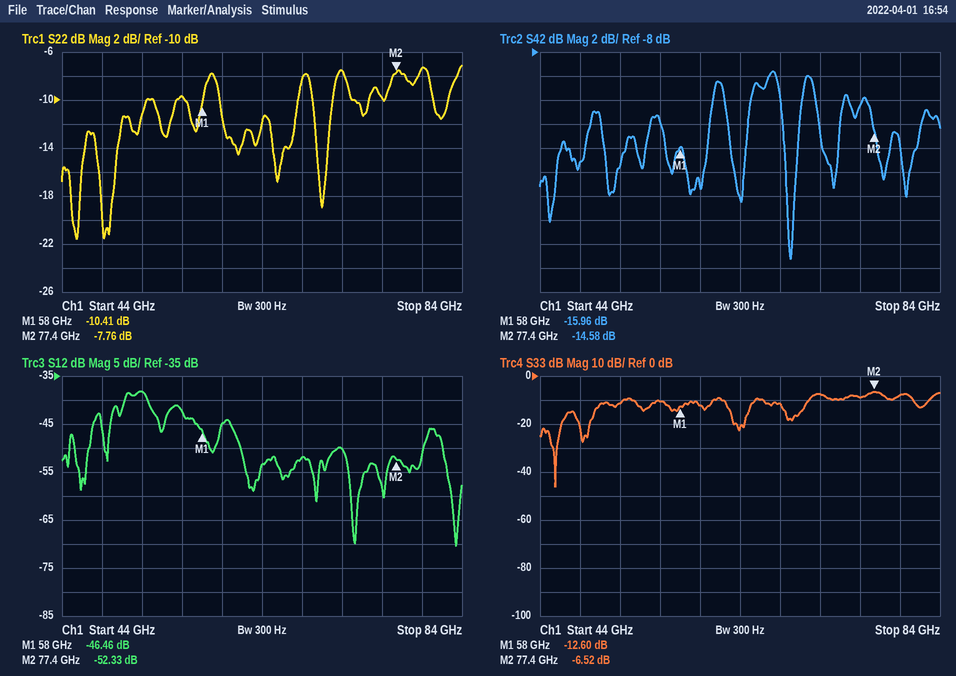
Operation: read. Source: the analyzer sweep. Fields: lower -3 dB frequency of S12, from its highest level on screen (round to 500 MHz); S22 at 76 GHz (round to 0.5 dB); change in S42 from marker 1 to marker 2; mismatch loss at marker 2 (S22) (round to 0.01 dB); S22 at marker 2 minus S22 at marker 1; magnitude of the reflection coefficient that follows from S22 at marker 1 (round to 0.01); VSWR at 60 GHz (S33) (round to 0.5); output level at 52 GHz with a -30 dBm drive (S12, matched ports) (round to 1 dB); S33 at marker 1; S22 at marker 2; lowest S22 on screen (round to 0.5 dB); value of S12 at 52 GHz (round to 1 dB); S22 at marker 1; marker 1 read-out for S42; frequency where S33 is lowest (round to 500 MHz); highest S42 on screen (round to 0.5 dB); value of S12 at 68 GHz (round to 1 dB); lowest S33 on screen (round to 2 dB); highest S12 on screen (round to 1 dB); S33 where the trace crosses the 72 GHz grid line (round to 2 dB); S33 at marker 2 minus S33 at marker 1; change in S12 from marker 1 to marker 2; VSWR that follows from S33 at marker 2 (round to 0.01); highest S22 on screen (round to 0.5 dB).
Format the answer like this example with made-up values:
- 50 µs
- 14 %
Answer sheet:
- 50.0 GHz
- -10.0 dB
- 1.38 dB
- 0.80 dB
- 2.65 dB
- 0.30
- 1.5
- -68 dBm
- -12.60 dB
- -7.76 dB
- -21.5 dB
- -38 dB
- -10.41 dB
- -15.96 dB
- 45.5 GHz
- -9.5 dB
- -52 dB
- -46 dB
- -38 dB
- -8 dB
- 6.08 dB
- -5.87 dB
- 2.79
- -7.0 dB
